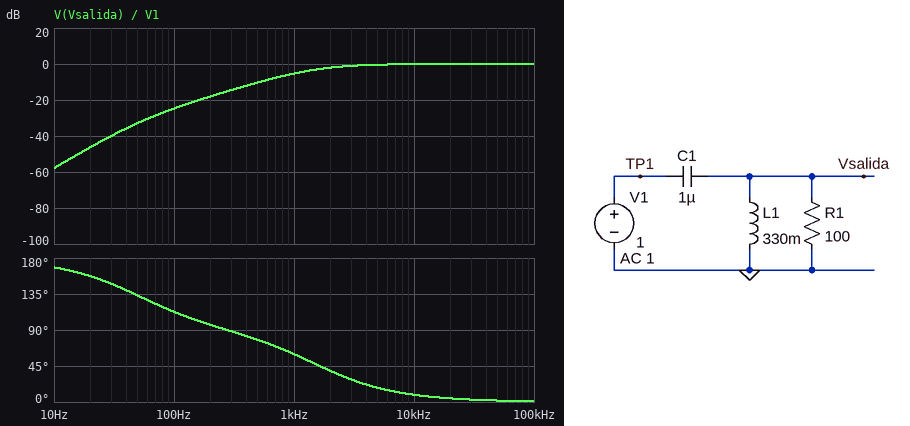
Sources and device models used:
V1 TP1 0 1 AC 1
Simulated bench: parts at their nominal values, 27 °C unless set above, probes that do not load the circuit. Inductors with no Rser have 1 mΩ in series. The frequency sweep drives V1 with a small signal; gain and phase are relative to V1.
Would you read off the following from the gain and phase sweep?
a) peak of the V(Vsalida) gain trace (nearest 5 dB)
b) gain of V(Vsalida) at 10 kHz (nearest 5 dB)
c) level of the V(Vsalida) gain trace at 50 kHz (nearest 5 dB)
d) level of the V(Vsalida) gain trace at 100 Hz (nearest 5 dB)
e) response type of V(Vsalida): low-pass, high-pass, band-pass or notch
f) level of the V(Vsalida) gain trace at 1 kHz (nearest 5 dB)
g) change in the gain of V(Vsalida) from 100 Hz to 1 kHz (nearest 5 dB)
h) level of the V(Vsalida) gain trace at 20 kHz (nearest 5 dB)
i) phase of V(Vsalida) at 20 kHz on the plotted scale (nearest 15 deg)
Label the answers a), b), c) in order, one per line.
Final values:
a) 0 dB
b) 0 dB
c) 0 dB
d) -25 dB
e) high-pass
f) -5 dB
g) 20 dB
h) 0 dB
i) 0 deg
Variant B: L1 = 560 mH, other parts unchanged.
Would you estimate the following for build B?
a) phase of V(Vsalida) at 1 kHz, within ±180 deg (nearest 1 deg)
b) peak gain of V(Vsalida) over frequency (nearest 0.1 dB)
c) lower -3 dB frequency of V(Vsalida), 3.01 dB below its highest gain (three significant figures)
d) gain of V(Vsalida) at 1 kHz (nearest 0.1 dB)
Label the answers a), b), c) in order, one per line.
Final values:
a) 59 deg
b) 0 dB
c) 1.56 kHz
d) -5.4 dB
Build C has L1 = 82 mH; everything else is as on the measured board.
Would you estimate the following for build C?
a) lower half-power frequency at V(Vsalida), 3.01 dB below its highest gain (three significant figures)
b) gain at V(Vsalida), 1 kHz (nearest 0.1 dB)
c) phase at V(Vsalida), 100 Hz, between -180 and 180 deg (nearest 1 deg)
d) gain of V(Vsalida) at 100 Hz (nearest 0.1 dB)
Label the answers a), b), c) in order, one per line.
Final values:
a) 1.40 kHz
b) -4.8 dB
c) 152 deg
d) -30.6 dB
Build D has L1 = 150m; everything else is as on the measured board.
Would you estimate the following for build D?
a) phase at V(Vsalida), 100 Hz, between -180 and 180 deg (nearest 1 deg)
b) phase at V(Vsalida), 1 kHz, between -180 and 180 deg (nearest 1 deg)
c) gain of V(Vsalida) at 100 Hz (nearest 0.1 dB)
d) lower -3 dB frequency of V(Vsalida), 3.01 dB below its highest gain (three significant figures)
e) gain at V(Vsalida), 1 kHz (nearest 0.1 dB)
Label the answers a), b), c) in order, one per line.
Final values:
a) 135 deg
b) 62 deg
c) -27.0 dB
d) 1.49 kHz
e) -5.1 dB
